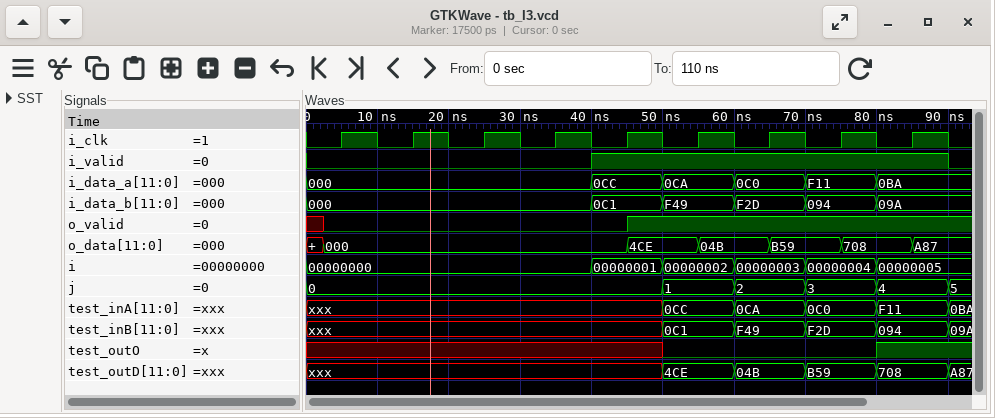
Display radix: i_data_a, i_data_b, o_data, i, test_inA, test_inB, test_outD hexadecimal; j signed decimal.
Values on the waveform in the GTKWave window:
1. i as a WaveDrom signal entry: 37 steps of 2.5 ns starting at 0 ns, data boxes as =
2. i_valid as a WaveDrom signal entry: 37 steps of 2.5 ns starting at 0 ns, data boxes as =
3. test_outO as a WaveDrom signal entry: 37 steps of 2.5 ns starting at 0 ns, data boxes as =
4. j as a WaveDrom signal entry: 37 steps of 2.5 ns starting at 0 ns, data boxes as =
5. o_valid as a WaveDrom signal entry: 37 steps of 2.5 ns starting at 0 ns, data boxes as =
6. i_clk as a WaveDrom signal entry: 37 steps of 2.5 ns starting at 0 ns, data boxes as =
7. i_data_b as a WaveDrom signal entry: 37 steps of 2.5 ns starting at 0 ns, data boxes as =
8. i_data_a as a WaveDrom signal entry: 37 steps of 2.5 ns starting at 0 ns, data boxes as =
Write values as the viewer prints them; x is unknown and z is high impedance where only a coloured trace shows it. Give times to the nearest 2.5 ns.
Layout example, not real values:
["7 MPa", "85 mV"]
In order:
["{name: 'i', wave: '=...............=...=...=...=...=....', data: '00000000 00000001 00000002 00000003 00000004 00000005'}", "{name: 'i_valid', wave: '0...............1...................0'}", "{name: 'test_outO', wave: 'x...................0...........1....'}", "{name: 'j', wave: '=...................=...=...=...=...=', data: '0 1 2 3 4 5'}", "{name: 'o_valid', wave: 'x0................1..................'}", "{name: 'i_clk', wave: '0.1.0.1.0.1.0.1.0.1.0.1.0.1.0.1.0.1.0'}", "{name: 'i_data_b', wave: '=...............=...=...=...=...=....', data: '000 0C1 F49 F2D 094 09A'}", "{name: 'i_data_a', wave: '=...............=...=...=...=...=....', data: '000 0CC 0CA 0C0 F11 0BA'}"]
